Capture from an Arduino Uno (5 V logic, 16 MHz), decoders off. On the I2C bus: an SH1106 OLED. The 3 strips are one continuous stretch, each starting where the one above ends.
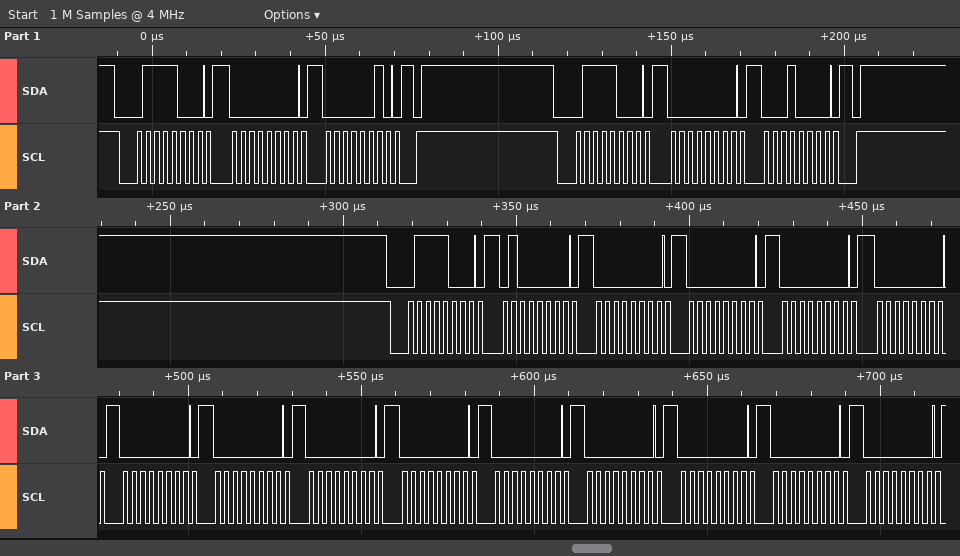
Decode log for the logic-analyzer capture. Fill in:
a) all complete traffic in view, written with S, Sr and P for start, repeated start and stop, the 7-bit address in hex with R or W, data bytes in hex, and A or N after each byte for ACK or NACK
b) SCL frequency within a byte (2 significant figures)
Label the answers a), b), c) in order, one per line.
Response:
a) S 3CW A 00 A 02 A P S 3CW A 00 A 10 A P S 3CW A 40 A 00 A 00 A 00 A 00 A 00 A 00 A 00 A 00 A 00 A 00 A 00 A 00 A 00 A
b) 400 kHz
